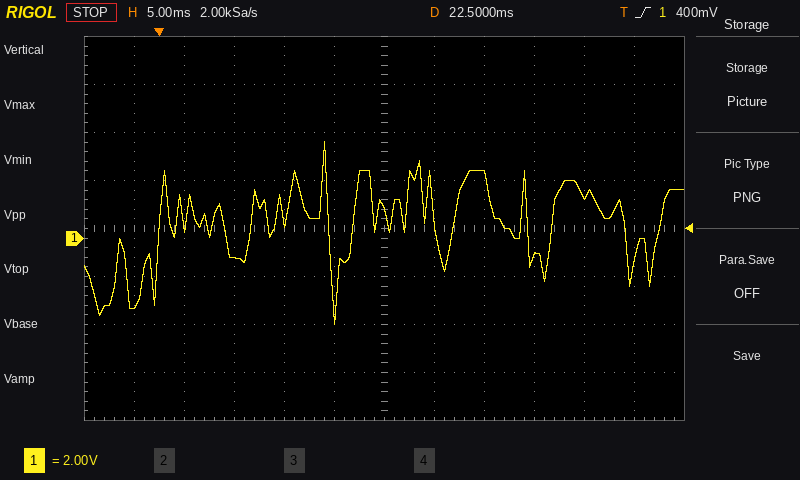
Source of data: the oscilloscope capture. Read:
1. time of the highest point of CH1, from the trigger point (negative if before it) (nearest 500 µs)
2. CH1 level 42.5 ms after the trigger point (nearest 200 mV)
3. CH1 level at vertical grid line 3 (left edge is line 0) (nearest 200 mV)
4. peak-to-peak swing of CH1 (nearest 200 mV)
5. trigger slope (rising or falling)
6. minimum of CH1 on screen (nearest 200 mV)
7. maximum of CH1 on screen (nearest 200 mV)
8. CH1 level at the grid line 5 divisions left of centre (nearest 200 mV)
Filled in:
+16.5 ms
1.8 V
-800 mV
7.6 V
rising
-3.6 V
4.0 V
-2.8 V
